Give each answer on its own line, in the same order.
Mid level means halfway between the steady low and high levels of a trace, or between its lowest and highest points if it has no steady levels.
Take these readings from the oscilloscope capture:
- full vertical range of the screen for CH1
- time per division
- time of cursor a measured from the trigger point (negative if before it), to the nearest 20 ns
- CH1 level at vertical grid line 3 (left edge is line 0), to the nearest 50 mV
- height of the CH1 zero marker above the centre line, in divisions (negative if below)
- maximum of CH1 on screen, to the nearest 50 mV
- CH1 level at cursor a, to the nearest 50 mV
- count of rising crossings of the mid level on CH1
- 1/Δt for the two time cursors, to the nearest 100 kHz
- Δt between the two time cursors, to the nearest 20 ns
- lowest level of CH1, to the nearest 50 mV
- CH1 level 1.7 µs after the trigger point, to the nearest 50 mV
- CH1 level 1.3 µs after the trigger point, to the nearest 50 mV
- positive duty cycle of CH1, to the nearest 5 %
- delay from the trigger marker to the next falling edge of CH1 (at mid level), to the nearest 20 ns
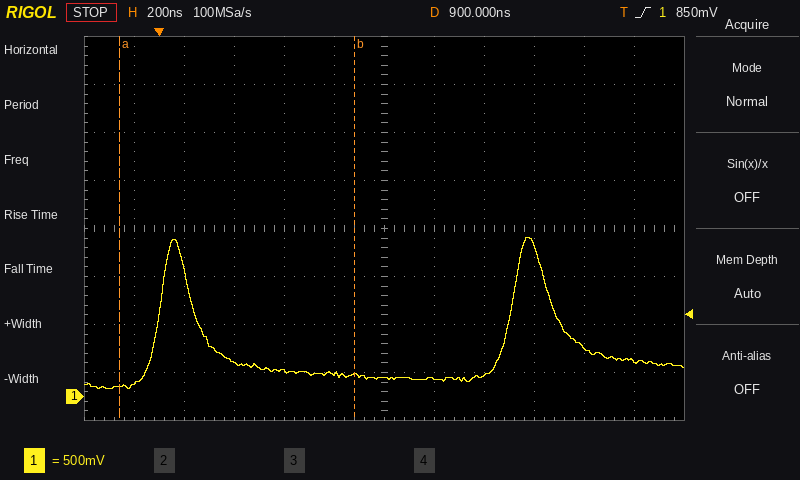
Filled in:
4 V
200 ns
-160 ns
350 mV
-3.5 div
1.65 V
100 mV
2
1.1 MHz
940 ns
100 mV
500 mV
200 mV
10 %
140 ns
